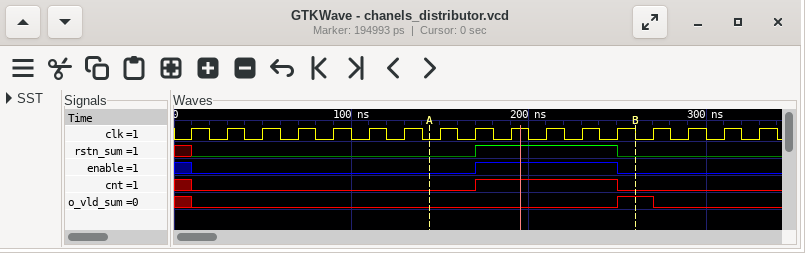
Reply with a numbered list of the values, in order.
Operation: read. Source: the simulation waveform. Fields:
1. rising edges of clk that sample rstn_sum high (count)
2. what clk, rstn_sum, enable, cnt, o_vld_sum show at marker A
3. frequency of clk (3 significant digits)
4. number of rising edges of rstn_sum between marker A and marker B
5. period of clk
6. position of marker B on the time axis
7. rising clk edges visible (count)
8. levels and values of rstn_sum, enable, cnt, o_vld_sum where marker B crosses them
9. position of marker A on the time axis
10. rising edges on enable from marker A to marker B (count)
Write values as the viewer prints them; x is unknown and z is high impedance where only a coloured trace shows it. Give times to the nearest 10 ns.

1. 4
2. clk=0, rstn_sum=0, enable=0, cnt=0, o_vld_sum=0
3. 50.0 MHz
4. 1
5. 20 ns
6. 260 ns
7. 17
8. rstn_sum=0, enable=0, cnt=0, o_vld_sum=1
9. 140 ns
10. 1
